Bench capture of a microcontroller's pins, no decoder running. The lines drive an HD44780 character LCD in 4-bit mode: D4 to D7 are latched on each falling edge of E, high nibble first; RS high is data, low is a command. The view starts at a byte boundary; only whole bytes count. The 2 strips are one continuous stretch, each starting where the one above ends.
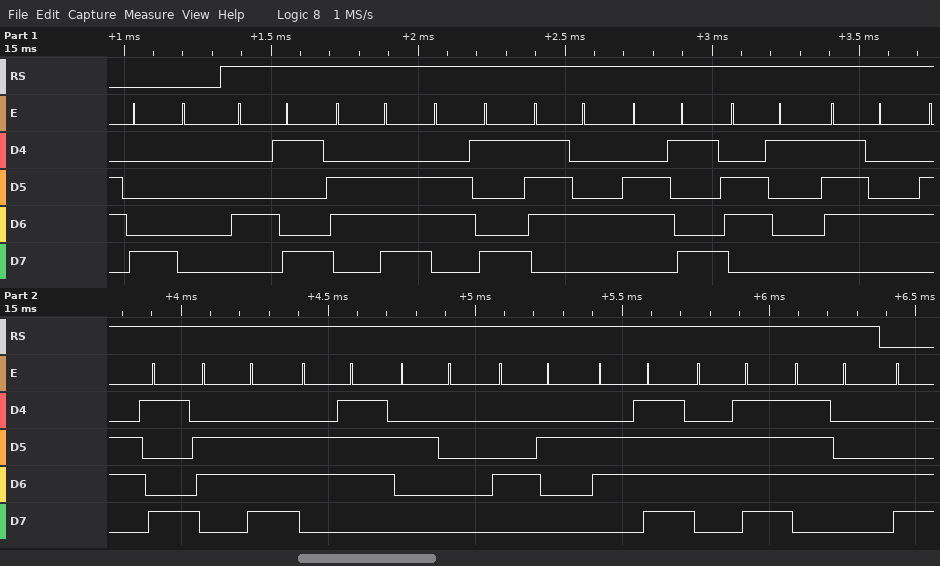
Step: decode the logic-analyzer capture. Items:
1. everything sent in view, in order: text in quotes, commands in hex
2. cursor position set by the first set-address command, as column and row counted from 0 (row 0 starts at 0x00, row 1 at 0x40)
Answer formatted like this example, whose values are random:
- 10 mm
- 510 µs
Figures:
- 0x80 "Initiating Boot"
- column 0, row 0
